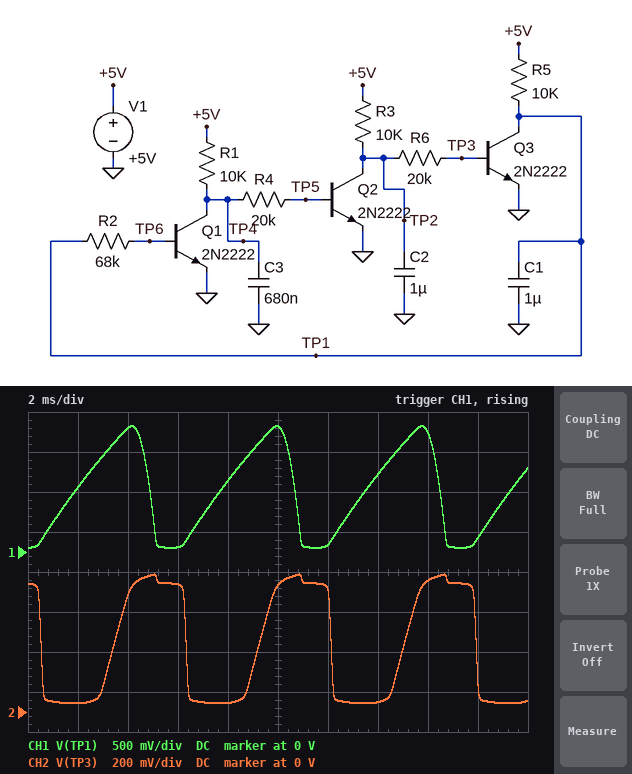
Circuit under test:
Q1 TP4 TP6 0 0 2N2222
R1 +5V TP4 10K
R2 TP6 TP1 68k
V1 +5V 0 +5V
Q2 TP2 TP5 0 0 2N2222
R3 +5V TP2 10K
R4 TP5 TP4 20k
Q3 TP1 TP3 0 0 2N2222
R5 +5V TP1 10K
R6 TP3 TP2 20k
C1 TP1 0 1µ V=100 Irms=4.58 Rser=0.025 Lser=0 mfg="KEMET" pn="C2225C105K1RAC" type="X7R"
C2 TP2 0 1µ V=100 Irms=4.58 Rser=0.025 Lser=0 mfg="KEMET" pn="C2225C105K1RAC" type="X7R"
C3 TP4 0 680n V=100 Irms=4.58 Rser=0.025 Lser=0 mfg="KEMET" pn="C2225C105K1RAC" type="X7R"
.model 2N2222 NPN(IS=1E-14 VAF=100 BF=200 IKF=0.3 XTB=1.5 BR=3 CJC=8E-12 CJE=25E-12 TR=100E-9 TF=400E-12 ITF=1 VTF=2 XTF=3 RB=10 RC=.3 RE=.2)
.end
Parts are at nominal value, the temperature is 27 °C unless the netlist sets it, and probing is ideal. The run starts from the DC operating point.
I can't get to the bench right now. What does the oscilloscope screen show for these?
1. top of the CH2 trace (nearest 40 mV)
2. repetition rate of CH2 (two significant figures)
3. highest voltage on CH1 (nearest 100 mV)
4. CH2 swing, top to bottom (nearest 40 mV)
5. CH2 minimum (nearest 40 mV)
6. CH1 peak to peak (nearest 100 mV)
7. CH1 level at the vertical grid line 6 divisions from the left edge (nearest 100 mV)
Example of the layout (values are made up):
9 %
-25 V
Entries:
680 mV
170 Hz
1.6 V
640 mV
40 mV
1.5 V
100 mV
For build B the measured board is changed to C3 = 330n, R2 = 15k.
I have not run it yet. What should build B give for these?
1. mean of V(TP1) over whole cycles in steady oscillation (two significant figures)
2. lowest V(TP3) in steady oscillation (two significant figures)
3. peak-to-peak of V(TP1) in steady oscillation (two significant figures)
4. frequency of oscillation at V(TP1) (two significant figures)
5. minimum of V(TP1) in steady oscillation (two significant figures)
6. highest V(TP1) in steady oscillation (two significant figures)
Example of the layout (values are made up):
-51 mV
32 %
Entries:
700 mV
36 mV
1.2 V
230 Hz
61 mV
1.3 V
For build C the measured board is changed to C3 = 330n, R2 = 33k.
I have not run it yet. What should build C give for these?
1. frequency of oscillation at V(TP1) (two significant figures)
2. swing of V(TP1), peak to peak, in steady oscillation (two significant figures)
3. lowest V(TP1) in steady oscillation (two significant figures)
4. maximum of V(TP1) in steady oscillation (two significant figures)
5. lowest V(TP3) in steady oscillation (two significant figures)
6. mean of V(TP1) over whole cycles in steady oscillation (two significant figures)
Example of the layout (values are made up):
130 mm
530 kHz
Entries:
220 Hz
1.3 V
61 mV
1.4 V
35 mV
750 mV
